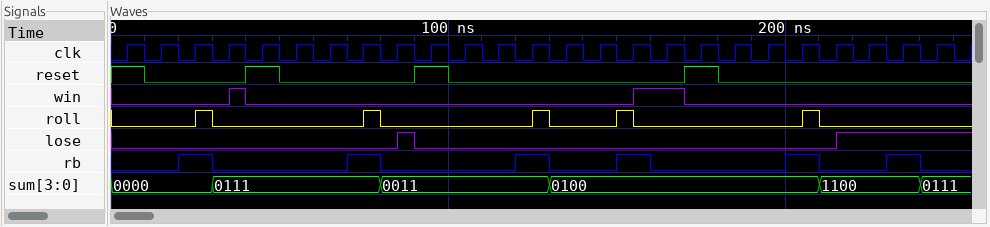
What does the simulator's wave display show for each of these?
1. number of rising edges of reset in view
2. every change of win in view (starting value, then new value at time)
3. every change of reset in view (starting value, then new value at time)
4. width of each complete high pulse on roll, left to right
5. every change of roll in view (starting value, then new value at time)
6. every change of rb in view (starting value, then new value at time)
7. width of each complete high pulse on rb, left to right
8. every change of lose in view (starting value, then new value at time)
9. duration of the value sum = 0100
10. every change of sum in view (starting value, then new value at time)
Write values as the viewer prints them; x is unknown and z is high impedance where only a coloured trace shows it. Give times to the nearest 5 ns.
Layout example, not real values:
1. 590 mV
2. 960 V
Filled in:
1. 3
2. 0, 1 at 35 ns, 0 at 40 ns, 1 at 155 ns, 0 at 170 ns
3. 1, 0 at 10 ns, 1 at 40 ns, 0 at 50 ns, 1 at 90 ns, 0 at 100 ns, 1 at 170 ns, 0 at 180 ns
4. 5 ns, 5 ns, 5 ns, 5 ns, 5 ns
5. 0, 1 at 25 ns, 0 at 30 ns, 1 at 75 ns, 0 at 80 ns, 1 at 125 ns, 0 at 130 ns, 1 at 150 ns, 0 at 155 ns, 1 at 205 ns, 0 at 210 ns
6. 0, 1 at 20 ns, 0 at 30 ns, 1 at 70 ns, 0 at 80 ns, 1 at 120 ns, 0 at 130 ns, 1 at 150 ns, 0 at 160 ns, 1 at 200 ns, 0 at 210 ns, 1 at 230 ns, 0 at 240 ns
7. 10 ns, 10 ns, 10 ns, 10 ns, 10 ns, 10 ns
8. 0, 1 at 85 ns, 0 at 90 ns, 1 at 215 ns
9. 80 ns
10. 0000, 0111 at 30 ns, 0011 at 80 ns, 0100 at 130 ns, 1100 at 210 ns, 0111 at 240 ns
